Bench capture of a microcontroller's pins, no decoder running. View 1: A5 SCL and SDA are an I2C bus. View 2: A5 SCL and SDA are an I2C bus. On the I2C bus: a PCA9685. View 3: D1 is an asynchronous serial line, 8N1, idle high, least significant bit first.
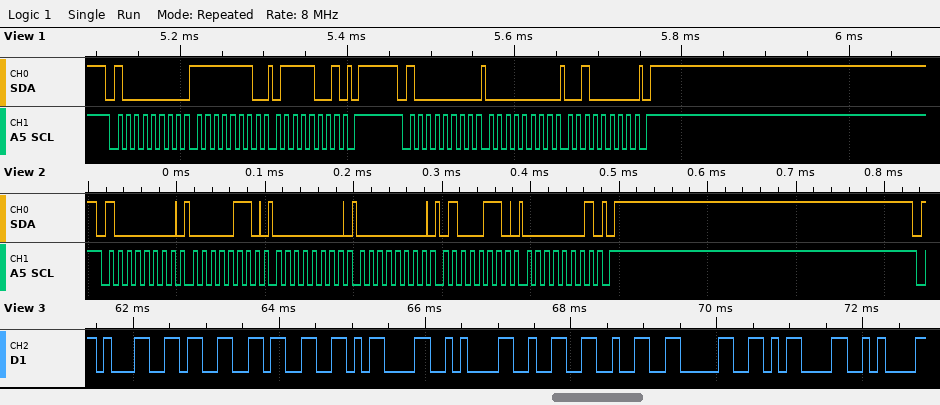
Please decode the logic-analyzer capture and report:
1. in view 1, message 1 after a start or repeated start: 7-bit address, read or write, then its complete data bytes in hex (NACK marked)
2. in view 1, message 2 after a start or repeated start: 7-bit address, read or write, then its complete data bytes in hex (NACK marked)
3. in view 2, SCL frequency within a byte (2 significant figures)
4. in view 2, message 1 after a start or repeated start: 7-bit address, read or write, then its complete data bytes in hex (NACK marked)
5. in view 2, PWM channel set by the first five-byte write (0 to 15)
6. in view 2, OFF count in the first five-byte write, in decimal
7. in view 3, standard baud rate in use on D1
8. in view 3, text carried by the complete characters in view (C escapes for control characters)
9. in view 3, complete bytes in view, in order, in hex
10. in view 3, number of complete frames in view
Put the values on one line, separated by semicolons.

0x40 write: FE 79; 0x40 write: 00 20; 100 kHz; 0x40 write: 06 00 00 46 01; 0; 326; 9600 baud; "133\r\n220\r\n"; 31 33 33 0D 0A 32 32 30 0D 0A; 10
